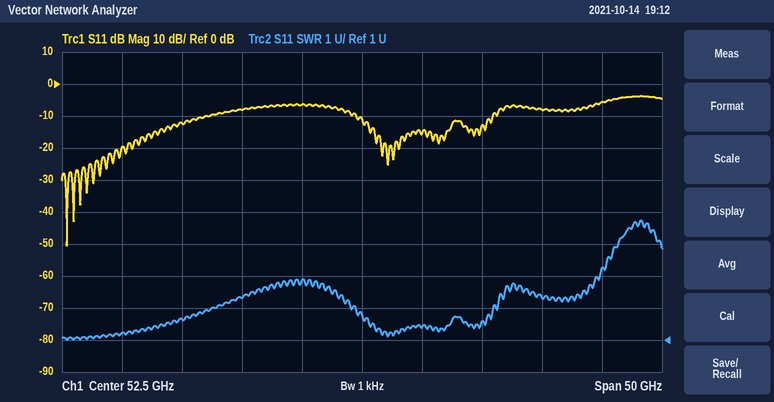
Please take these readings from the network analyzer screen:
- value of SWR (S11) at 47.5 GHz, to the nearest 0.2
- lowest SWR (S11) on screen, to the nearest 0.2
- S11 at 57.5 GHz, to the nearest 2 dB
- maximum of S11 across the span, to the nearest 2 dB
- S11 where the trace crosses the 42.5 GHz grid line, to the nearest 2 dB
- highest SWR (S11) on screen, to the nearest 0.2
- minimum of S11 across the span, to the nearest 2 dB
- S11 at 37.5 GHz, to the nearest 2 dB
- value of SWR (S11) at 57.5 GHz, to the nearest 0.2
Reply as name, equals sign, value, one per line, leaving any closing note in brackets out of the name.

value of SWR (S11) at 47.5 GHz, to the nearest 0.2 = 2.8
lowest SWR (S11) on screen, to the nearest 0.2 = 1.0
S11 at 57.5 GHz, to the nearest 2 dB = -16 dB
maximum of S11 across the span, to the nearest 2 dB = -4 dB
S11 where the trace crosses the 42.5 GHz grid line, to the nearest 2 dB = -8 dB
highest SWR (S11) on screen, to the nearest 0.2 = 4.8
minimum of S11 across the span, to the nearest 2 dB = -50 dB
S11 at 37.5 GHz, to the nearest 2 dB = -12 dB
value of SWR (S11) at 57.5 GHz, to the nearest 0.2 = 1.4
